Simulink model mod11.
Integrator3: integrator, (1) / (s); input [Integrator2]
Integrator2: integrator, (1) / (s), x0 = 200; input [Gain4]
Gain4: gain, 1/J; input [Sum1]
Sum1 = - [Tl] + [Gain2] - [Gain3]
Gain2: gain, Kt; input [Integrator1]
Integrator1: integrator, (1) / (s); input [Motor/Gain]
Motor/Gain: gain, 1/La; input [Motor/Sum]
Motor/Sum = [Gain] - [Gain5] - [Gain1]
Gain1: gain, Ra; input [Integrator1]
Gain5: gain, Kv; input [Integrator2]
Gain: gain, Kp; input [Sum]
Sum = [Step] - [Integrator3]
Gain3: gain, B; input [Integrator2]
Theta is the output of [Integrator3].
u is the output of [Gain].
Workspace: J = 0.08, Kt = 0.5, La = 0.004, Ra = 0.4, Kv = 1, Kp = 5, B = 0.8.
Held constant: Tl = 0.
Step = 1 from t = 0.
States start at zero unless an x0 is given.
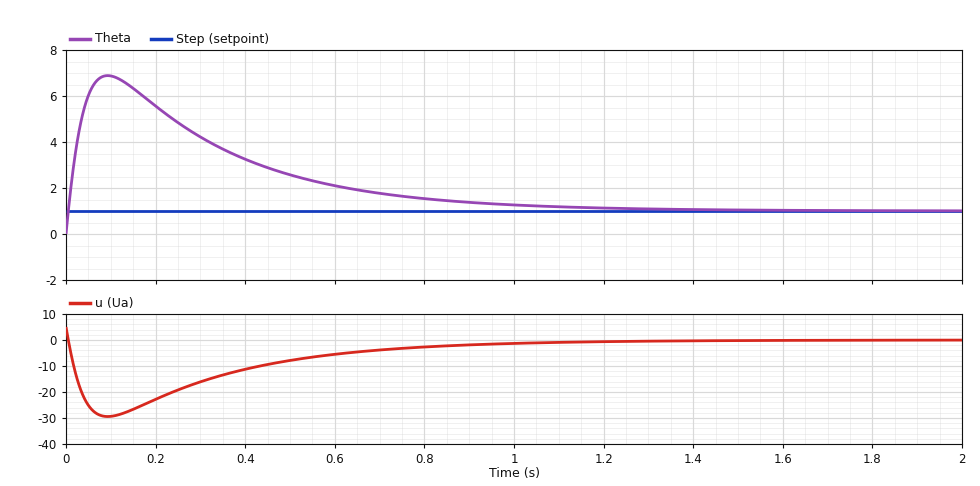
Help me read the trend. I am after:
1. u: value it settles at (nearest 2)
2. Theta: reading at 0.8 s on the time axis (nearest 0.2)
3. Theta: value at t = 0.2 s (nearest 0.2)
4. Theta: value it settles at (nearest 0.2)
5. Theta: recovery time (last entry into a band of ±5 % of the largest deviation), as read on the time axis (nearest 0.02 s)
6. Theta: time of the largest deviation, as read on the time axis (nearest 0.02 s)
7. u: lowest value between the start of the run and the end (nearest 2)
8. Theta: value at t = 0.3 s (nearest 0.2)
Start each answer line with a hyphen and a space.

- 0
- 1.6
- 5.6
- 1.0
- 0.92 s
- 0.10 s
- -30
- 4.2
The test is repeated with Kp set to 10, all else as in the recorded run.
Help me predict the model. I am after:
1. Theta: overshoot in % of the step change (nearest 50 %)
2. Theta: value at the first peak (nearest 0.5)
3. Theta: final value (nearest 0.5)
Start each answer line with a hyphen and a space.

- 550 %
- 6.5
- 1.0
